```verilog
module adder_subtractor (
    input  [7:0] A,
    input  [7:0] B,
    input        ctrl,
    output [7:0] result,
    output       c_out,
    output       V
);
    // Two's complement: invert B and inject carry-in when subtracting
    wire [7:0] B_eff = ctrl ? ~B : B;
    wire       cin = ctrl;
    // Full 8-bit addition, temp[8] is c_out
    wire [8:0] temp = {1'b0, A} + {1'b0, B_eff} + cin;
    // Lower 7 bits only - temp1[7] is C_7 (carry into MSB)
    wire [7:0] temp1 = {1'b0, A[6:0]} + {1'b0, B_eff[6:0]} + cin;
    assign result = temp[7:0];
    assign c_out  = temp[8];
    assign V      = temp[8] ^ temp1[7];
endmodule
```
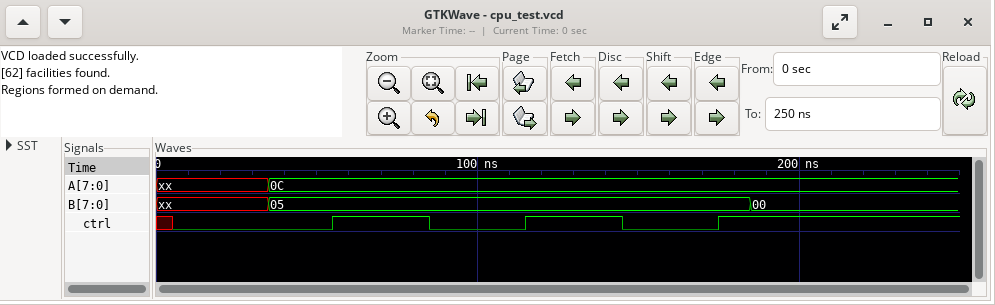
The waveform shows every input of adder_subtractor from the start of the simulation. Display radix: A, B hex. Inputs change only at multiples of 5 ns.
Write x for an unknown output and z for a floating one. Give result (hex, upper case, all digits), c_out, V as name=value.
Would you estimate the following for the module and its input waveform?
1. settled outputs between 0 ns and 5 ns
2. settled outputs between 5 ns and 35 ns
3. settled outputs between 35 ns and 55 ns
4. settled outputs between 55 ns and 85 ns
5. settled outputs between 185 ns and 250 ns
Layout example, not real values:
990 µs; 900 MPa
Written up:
result=x, c_out=x, V=x; result=x, c_out=x, V=x; result=11, c_out=0, V=0; result=07, c_out=1, V=0; result=0C, c_out=1, V=0
